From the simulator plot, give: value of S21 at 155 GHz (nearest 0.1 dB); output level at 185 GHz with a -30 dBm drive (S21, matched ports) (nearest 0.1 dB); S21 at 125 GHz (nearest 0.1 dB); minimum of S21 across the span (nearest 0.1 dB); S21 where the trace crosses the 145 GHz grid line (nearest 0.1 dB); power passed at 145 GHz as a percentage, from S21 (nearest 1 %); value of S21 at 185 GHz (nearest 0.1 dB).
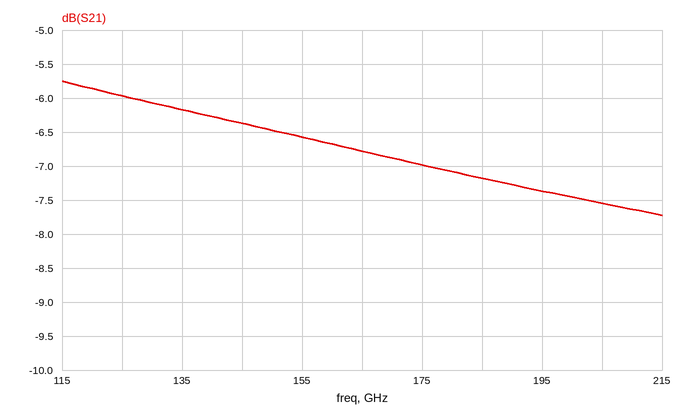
-6.6 dB
-37.2 dBm
-6.0 dB
-7.7 dB
-6.4 dB
23 %
-7.2 dB
